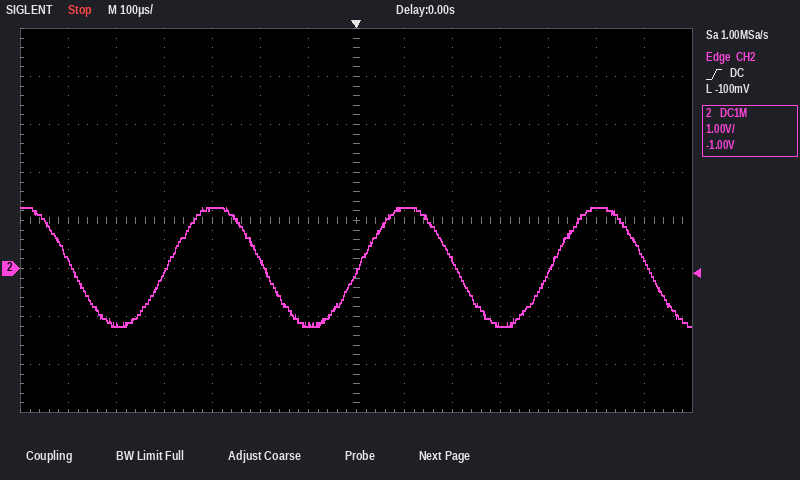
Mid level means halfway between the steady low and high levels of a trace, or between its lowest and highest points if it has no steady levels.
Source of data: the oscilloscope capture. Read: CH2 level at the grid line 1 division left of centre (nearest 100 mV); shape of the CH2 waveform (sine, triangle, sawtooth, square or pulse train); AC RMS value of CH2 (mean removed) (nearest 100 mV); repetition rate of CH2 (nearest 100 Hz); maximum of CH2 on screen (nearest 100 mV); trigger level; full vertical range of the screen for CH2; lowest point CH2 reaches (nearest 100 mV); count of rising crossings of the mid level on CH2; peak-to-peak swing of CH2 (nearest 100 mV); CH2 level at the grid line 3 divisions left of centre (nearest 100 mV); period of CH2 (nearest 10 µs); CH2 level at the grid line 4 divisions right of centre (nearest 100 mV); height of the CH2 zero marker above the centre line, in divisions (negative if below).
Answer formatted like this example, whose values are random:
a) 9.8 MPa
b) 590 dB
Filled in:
a) -1.2 V
b) sine
c) 900 mV
d) 2.5 kHz
e) 1.3 V
f) -100 mV
g) 8 V
h) -1.2 V
i) 3
j) 2.5 V
k) 1.3 V
l) 400 µs
m) -100 mV
n) -1.0 div
